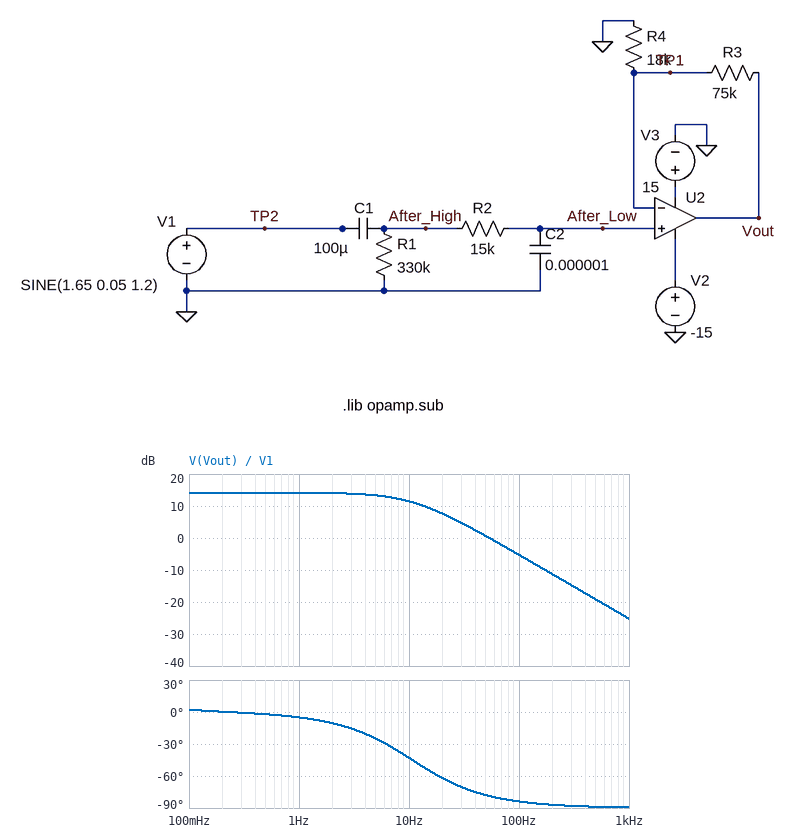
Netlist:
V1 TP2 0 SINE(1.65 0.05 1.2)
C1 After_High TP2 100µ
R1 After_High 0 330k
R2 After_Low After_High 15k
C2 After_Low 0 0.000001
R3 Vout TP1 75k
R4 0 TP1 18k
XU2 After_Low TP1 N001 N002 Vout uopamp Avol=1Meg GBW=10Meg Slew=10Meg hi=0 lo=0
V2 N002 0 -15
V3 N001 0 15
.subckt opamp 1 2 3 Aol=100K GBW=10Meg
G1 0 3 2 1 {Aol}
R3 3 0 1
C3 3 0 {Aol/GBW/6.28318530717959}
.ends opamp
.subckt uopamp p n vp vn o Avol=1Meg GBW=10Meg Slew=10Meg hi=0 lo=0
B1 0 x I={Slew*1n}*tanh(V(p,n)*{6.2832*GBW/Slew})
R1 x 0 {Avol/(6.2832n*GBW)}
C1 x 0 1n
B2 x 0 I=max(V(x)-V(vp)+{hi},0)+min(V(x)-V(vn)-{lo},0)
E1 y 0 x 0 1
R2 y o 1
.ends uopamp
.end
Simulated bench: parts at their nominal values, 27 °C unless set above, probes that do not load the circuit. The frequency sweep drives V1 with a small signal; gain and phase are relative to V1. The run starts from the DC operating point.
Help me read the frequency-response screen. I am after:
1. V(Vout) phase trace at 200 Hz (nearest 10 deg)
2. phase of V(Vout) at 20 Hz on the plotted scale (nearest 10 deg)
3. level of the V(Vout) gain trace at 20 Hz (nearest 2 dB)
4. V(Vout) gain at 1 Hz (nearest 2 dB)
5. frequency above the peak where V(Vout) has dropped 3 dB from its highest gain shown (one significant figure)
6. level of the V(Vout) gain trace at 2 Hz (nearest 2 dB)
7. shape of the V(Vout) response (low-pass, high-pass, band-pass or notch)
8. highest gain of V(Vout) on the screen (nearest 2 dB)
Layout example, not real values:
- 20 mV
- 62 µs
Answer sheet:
- -90 deg
- -60 deg
- 8 dB
- 14 dB
- 10 Hz
- 14 dB
- low-pass
- 14 dB
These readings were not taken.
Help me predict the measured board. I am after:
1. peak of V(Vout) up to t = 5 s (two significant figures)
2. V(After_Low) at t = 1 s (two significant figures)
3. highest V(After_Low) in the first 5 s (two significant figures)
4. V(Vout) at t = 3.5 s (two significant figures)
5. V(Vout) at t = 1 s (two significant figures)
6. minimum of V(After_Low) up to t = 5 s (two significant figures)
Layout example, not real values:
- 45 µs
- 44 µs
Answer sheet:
- 250 mV
- 45 mV
- 49 mV
- 230 mV
- 230 mV
- -49 mV
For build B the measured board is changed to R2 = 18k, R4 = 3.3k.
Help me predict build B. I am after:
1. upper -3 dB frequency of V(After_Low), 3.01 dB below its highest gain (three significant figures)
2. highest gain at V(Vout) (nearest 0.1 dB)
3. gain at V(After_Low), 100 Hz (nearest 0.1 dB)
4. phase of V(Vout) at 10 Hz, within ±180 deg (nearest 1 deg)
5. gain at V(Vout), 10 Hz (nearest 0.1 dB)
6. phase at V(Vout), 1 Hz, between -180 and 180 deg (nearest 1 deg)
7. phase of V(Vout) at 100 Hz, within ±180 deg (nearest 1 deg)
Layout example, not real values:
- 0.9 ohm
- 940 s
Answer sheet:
- 8.94 Hz
- 27.4 dB
- -21.1 dB
- -48 deg
- 23.9 dB
- -6 deg
- -85 deg
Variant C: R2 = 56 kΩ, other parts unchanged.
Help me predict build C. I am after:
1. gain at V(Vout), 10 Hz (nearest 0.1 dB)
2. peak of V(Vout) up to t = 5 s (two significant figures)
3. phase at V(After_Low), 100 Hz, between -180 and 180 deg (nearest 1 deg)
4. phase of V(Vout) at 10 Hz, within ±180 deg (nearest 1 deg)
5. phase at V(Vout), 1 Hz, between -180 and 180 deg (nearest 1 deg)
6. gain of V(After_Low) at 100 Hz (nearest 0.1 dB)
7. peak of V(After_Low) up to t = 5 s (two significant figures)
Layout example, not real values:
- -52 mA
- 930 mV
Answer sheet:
- 3.0 dB
- 240 mV
- -88 deg
- -74 deg
- -19 deg
- -30.9 dB
- 46 mV
